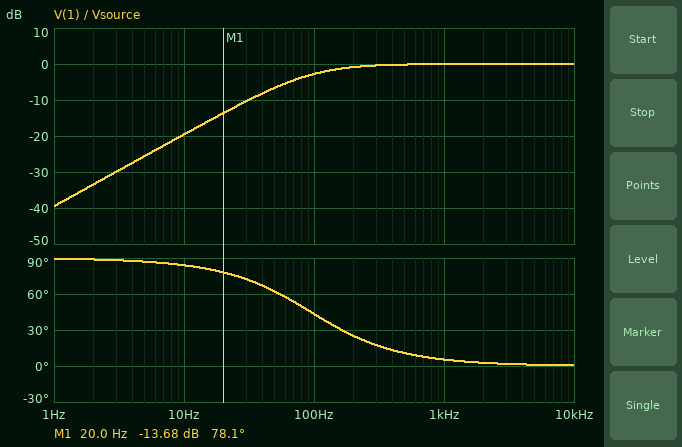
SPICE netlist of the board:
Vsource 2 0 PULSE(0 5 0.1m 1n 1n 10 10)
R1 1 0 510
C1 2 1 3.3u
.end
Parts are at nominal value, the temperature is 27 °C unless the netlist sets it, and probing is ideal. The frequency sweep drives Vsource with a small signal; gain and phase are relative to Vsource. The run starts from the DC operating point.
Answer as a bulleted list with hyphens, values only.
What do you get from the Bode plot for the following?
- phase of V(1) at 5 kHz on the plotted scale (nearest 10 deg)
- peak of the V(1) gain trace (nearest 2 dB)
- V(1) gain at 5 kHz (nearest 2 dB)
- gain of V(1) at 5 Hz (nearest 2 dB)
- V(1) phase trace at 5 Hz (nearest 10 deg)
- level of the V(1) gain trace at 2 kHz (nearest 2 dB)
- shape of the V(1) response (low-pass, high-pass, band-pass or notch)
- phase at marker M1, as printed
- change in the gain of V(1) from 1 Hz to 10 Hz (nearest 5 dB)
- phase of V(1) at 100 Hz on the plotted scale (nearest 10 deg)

- 0 deg
- 0 dB
- 0 dB
- -26 dB
- 90 deg
- 0 dB
- high-pass
- 78.1 deg
- 20 dB
- 40 deg
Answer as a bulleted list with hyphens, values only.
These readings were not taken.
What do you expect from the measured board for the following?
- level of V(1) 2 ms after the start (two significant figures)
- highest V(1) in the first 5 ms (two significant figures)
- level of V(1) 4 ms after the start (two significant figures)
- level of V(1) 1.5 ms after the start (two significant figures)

- 1.6 V
- 5.0 V
- 490 mV
- 2.2 V
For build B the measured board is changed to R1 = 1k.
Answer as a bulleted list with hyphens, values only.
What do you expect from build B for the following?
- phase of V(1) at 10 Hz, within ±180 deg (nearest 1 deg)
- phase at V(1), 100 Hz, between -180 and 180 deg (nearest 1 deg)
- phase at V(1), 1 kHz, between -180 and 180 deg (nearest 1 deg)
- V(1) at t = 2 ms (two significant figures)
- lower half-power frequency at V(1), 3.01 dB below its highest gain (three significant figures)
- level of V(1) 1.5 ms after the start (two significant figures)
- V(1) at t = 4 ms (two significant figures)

- 78 deg
- 26 deg
- 3 deg
- 2.8 V
- 48.2 Hz
- 3.3 V
- 1.5 V
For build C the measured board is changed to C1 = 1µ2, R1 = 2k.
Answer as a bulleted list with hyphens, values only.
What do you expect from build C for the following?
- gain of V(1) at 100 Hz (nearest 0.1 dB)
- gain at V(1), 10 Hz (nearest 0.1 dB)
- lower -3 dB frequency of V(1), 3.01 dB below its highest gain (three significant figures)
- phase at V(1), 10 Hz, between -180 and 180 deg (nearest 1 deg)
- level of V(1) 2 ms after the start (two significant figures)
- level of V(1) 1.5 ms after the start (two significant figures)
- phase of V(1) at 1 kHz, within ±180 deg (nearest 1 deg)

- -1.6 dB
- -16.5 dB
- 66.3 Hz
- 81 deg
- 2.3 V
- 2.8 V
- 4 deg
